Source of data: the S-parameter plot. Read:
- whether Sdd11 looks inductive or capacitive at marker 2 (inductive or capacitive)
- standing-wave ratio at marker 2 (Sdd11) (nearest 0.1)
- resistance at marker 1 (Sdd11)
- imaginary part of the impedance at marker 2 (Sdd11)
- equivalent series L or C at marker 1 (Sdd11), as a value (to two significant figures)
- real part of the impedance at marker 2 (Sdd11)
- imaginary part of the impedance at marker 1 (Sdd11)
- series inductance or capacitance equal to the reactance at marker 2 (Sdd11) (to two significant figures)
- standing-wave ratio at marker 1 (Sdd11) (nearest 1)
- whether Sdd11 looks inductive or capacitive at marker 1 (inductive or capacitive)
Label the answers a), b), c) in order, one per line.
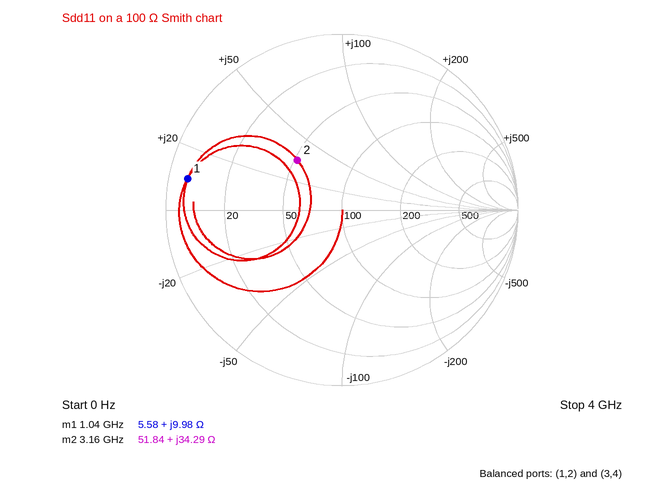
a) inductive
b) 2.2
c) 5.58 Ω
d) +34.29 Ω
e) 1.5 nH
f) 51.84 Ω
g) +9.98 Ω
h) 1.7 nH
i) 18
j) inductive
